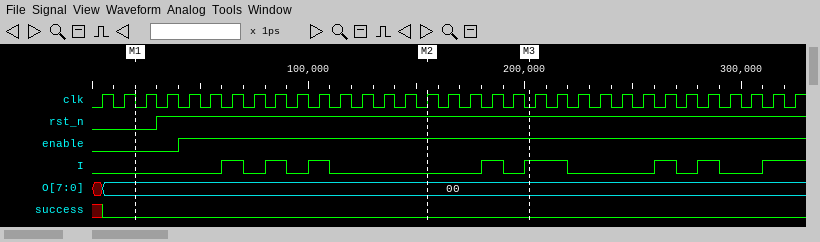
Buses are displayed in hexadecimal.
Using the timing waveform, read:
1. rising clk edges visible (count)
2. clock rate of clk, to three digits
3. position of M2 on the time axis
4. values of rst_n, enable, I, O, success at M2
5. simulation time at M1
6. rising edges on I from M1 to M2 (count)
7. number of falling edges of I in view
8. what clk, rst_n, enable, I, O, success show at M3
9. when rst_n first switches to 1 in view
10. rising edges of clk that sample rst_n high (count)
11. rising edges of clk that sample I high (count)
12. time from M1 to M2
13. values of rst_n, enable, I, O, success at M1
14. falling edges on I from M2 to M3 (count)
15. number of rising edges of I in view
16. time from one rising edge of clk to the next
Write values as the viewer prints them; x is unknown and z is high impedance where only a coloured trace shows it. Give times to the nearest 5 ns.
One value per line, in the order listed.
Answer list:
33
100 MHz
155 ns
rst_n=1, enable=1, I=0, O=00, success=0
20 ns
3
7
clk=0, rst_n=1, enable=1, I=1, O=00, success=0
30 ns
30
10
135 ns
rst_n=0, enable=0, I=0, O=00, success=0
1
8
10 ns
